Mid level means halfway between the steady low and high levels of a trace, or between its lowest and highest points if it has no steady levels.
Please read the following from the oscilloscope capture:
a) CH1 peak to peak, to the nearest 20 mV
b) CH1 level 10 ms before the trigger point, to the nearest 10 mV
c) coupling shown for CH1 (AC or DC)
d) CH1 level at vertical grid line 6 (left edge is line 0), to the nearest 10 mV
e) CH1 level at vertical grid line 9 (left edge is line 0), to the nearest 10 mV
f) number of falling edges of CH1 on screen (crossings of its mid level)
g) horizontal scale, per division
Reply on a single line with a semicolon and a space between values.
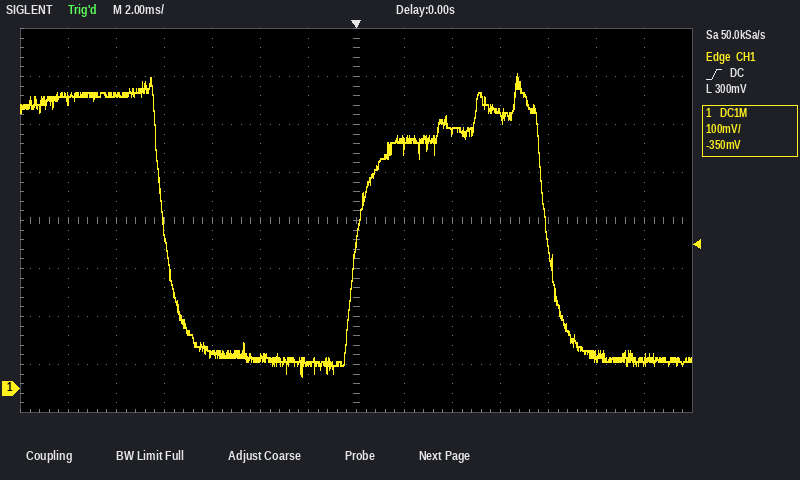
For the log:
640 mV; 610 mV; DC; 50 mV; 540 mV; 2; 2 ms
